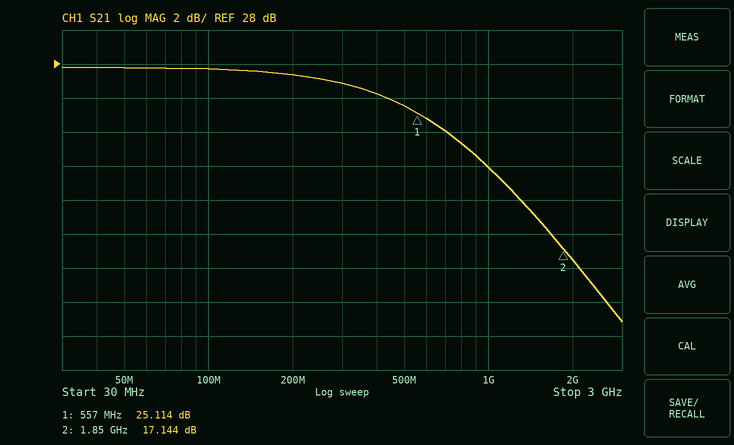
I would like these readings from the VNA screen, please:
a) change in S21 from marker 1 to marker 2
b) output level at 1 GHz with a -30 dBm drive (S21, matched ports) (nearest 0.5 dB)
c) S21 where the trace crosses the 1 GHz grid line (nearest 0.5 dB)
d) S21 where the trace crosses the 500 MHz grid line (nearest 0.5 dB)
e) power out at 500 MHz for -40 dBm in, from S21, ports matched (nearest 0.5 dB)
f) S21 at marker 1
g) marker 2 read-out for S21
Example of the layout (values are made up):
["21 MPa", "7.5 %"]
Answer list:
["-7.970 dB", "-8.0 dBm", "22.0 dB", "25.5 dB", "-14.5 dBm", "25.114 dB", "17.144 dB"]
